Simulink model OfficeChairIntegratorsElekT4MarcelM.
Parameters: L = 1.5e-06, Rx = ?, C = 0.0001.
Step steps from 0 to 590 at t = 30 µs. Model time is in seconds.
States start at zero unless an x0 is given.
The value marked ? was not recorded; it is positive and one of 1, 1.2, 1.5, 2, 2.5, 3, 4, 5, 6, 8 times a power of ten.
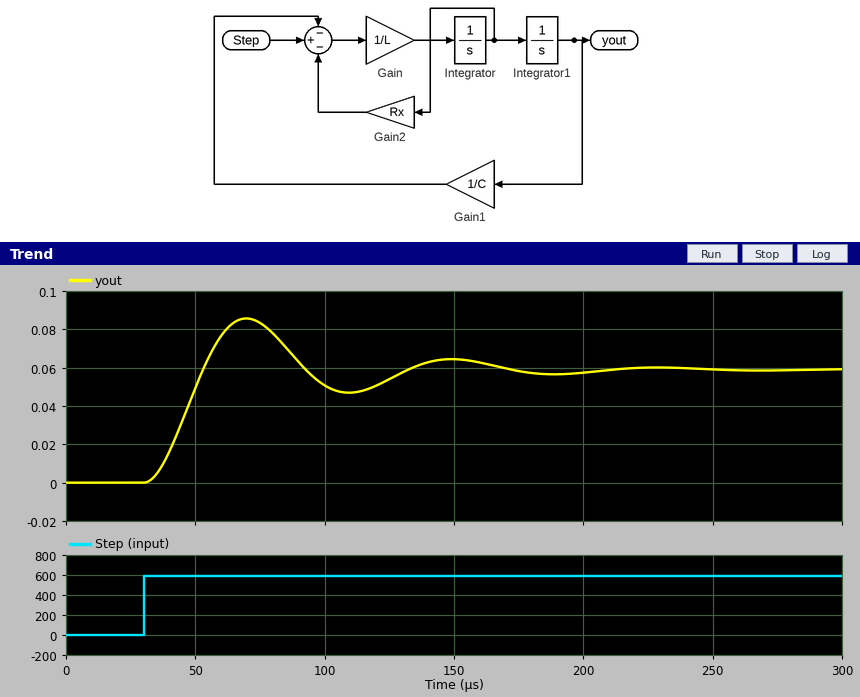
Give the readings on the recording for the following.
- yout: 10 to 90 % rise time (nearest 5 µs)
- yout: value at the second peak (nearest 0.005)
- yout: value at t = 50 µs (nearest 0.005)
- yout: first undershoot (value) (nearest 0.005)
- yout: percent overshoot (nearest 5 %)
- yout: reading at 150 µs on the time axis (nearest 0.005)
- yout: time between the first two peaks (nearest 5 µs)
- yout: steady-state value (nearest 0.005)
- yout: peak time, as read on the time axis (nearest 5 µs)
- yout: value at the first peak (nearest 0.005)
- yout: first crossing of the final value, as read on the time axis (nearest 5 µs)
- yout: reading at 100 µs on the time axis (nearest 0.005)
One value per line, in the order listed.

15 µs
0.065
0.050
0.045
45 %
0.065
80 µs
0.060
70 µs
0.085
55 µs
0.050
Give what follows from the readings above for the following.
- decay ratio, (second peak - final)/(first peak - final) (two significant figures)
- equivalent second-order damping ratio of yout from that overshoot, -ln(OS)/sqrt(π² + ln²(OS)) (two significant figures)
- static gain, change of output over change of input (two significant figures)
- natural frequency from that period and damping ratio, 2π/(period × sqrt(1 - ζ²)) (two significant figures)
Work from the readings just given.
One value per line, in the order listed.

0.20
0.25
0.00010
0.081 rad/µs
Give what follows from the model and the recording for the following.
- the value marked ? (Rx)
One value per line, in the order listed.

0.06
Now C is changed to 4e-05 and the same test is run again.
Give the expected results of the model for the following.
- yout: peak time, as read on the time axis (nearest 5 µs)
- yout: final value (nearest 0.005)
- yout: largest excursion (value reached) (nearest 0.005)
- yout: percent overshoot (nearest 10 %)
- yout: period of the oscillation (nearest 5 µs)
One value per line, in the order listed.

55 µs
0.025
0.040
60 %
50 µs
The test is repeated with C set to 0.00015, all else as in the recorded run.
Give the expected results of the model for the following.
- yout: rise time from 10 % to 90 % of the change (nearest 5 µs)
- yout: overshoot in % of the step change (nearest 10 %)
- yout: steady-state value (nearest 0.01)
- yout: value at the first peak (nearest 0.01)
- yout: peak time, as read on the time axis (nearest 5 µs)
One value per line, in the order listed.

20 µs
40 %
0.09
0.12
80 µs
